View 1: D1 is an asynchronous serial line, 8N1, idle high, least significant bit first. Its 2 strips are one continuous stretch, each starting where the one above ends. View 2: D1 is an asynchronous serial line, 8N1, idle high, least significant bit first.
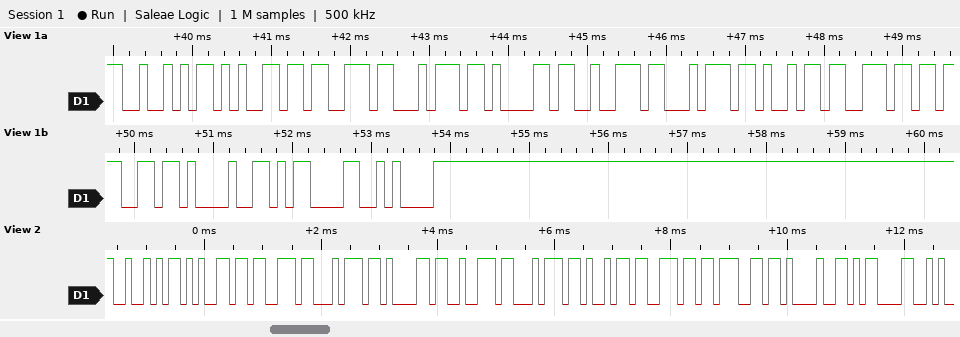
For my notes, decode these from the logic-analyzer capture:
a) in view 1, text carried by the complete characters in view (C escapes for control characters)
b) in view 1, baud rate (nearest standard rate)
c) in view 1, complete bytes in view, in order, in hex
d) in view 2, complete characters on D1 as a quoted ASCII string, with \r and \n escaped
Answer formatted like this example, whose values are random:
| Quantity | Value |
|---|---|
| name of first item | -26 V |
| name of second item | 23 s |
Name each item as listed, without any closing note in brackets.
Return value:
| Quantity | Value |
|---|---|
| in view 1, text carried by the complete characters in view | "Restarting!\r\n" |
| in view 1, baud rate | 9600 baud |
| in view 1, complete bytes in view, in order, in hex | 0x52 0x65 0x73 0x74 0x61 0x72 0x74 0x69 0x6E 0x67 0x21 0x0D 0x0A |
| in view 2, complete characters on D1 as a quoted ASCII string, with \r and \n escaped | "Restarting!\r" |
